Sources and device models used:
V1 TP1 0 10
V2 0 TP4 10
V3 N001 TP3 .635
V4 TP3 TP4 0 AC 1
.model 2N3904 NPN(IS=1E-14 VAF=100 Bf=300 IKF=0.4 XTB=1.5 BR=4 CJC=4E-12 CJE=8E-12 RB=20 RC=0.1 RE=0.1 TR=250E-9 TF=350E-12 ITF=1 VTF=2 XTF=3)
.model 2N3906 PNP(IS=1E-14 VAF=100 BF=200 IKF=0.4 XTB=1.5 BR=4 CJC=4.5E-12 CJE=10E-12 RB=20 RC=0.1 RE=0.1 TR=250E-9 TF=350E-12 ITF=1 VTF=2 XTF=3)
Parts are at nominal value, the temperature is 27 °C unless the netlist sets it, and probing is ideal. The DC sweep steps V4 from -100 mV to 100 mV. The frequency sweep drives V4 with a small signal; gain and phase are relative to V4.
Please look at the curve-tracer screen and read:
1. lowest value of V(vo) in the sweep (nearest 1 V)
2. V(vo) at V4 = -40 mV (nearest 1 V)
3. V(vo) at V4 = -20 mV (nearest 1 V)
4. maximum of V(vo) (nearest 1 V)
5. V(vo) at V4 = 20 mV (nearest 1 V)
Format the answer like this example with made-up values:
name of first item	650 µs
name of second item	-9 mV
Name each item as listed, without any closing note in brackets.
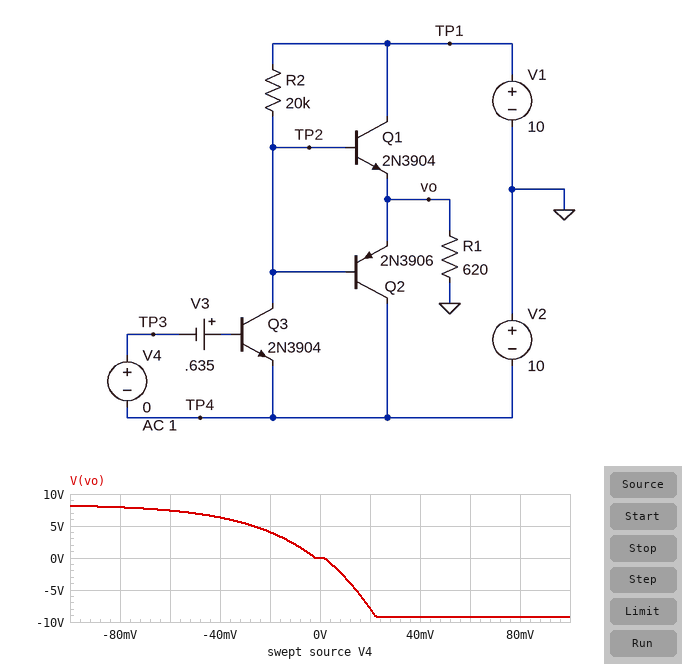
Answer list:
lowest value of V(vo) in the sweep	-9 V
V(vo) at V4 = -40 mV	6 V
V(vo) at V4 = -20 mV	4 V
maximum of V(vo)	8 V
V(vo) at V4 = 20 mV	-8 V
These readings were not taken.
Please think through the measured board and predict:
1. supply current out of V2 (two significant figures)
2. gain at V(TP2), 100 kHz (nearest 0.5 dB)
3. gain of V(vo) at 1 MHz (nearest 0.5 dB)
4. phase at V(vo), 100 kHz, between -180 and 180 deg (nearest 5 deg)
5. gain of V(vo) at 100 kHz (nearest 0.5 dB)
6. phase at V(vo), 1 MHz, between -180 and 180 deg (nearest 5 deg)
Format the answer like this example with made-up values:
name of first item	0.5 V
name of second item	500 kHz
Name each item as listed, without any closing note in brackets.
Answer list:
supply current out of V2	500 µA
gain at V(TP2), 100 kHz	50.5 dB
gain of V(vo) at 1 MHz	18.5 dB
phase at V(vo), 100 kHz, between -180 and 180 deg	-105 deg
gain of V(vo) at 100 kHz	7.5 dB
phase at V(vo), 1 MHz, between -180 and 180 deg	-160 deg
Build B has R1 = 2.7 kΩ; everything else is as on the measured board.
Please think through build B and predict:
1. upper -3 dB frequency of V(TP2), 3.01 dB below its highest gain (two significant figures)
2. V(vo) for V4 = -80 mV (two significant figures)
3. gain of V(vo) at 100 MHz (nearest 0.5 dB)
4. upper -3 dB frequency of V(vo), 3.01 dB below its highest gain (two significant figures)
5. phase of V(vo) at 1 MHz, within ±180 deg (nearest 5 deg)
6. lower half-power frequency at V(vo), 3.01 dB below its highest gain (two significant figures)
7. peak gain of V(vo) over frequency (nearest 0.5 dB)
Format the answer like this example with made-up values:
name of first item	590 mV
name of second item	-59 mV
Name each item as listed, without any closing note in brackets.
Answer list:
upper -3 dB frequency of V(TP2), 3.01 dB below its highest gain	340 kHz
V(vo) for V4 = -80 mV	8.6 V
gain of V(vo) at 100 MHz	14.0 dB
upper -3 dB frequency of V(vo), 3.01 dB below its highest gain	15 MHz
phase of V(vo) at 1 MHz, within ±180 deg	-165 deg
lower half-power frequency at V(vo), 3.01 dB below its highest gain	320 kHz
peak gain of V(vo) over frequency	31.0 dB
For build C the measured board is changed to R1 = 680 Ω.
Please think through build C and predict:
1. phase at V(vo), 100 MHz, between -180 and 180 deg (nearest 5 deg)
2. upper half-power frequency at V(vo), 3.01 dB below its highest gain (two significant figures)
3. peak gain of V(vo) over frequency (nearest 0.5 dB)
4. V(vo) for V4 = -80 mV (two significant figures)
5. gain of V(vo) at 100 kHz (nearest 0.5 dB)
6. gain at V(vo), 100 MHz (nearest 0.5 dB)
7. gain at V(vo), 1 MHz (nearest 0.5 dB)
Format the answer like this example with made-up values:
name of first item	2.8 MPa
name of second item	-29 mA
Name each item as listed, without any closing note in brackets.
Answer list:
phase at V(vo), 100 MHz, between -180 and 180 deg	100 deg
upper half-power frequency at V(vo), 3.01 dB below its highest gain	53 MHz
peak gain of V(vo) over frequency	19.5 dB
V(vo) for V4 = -80 mV	8.0 V
gain of V(vo) at 100 kHz	8.5 dB
gain at V(vo), 100 MHz	13.0 dB
gain at V(vo), 1 MHz	19.0 dB
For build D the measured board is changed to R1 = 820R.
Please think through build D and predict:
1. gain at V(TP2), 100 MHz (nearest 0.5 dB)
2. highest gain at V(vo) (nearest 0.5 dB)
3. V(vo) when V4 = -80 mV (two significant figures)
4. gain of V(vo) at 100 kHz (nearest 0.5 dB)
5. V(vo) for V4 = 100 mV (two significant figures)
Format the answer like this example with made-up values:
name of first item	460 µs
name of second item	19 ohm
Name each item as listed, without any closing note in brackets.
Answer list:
gain at V(TP2), 100 MHz	13.5 dB
highest gain at V(vo)	21.0 dB
V(vo) when V4 = -80 mV	8.1 V
gain of V(vo) at 100 kHz	10.0 dB
V(vo) for V4 = 100 mV	-9.3 V
